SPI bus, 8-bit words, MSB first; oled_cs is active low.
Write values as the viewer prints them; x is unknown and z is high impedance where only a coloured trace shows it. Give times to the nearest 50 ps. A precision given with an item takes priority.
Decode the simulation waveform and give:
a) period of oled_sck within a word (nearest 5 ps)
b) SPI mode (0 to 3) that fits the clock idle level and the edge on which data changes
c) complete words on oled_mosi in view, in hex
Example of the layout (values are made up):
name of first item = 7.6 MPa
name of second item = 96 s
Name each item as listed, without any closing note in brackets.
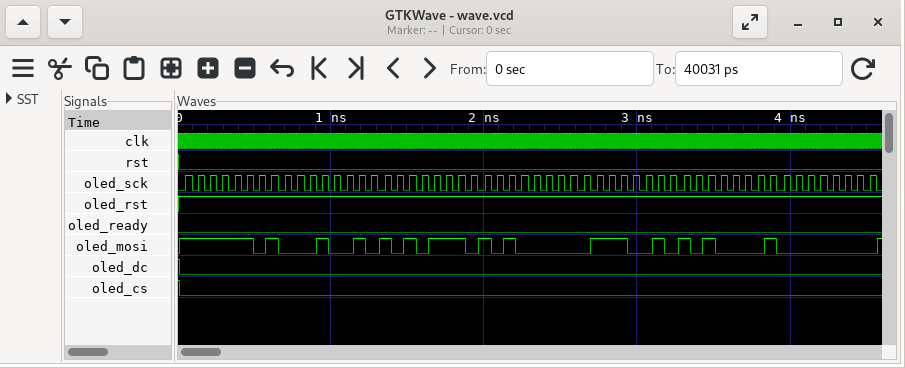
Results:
period of oled_sck within a word = 80 ps
SPI mode (0 to 3) that fits the clock idle level and the edge on which data changes = 0
complete words on oled_mosi in view, in hex = FD, 12, AE, A0, 72, A1, 00
